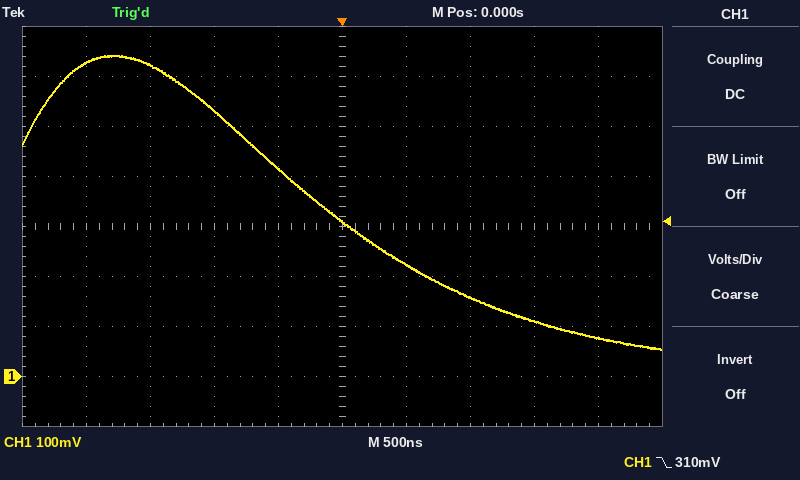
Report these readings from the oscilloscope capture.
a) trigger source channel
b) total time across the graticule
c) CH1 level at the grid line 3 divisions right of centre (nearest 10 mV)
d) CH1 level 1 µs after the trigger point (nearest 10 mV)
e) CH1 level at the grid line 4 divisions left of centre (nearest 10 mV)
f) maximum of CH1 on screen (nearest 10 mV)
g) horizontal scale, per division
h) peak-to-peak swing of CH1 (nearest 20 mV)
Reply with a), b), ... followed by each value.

a) CH1
b) 5 µs
c) 110 mV
d) 160 mV
e) 630 mV
f) 640 mV
g) 500 ns
h) 580 mV
